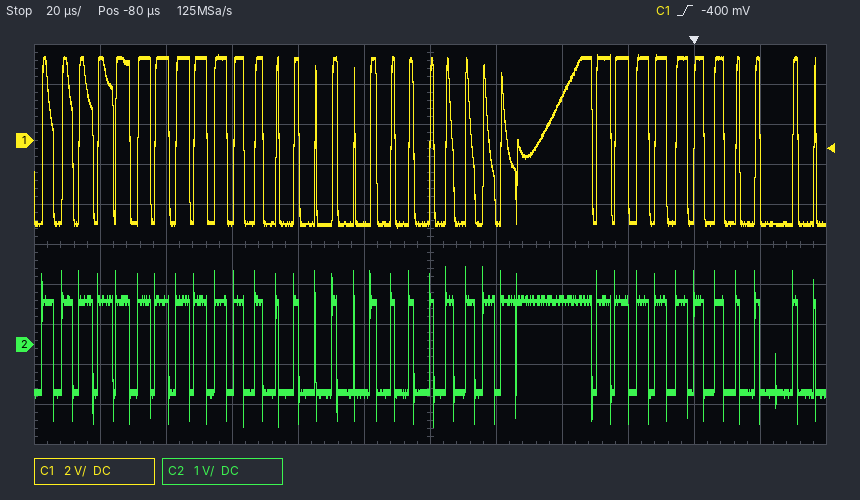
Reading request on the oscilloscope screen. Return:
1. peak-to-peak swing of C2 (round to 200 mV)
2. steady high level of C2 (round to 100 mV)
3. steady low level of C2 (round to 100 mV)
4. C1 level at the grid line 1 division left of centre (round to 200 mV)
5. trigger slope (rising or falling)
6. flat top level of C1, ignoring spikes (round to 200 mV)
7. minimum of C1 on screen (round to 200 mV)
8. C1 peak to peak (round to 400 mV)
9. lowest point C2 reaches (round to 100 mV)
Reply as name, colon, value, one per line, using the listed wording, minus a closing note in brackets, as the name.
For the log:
peak-to-peak swing of C2: 4.0 V
steady high level of C2: 1.1 V
steady low level of C2: -1.2 V
C1 level at the grid line 1 division left of centre: -4.2 V
trigger slope: rising
flat top level of C1, ignoring spikes: 4.2 V
minimum of C1 on screen: -4.4 V
C1 peak to peak: 8.8 V
lowest point C2 reaches: -2.1 V
